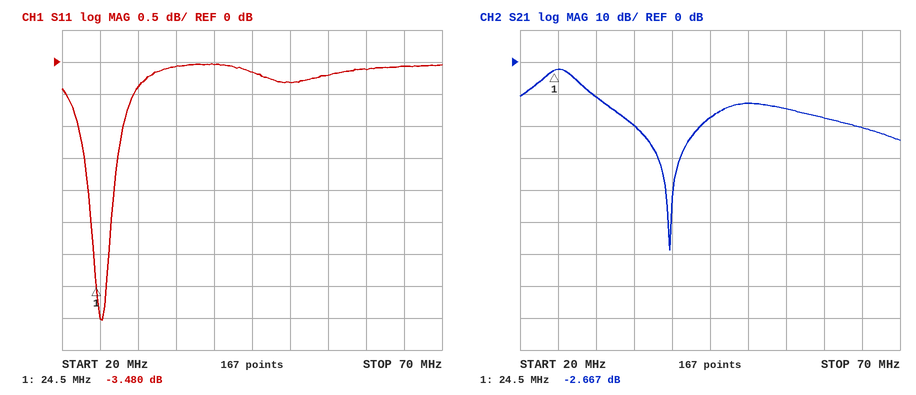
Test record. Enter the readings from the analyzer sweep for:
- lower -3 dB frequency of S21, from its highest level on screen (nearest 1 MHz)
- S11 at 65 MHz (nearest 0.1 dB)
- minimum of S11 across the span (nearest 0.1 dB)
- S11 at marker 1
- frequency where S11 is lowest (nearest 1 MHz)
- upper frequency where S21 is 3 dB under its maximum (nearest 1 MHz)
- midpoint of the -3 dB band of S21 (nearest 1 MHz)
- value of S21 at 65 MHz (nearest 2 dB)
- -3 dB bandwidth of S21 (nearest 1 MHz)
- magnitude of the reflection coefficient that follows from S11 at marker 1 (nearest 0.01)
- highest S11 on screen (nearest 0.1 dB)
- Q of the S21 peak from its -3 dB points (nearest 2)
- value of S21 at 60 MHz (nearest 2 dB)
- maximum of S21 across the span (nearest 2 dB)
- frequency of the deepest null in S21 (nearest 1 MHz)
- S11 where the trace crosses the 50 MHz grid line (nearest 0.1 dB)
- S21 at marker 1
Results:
23 MHz
-0.1 dB
-4.0 dB
-3.480 dB
25 MHz
27 MHz
25 MHz
-20 dB
4 MHz
0.67
0.0 dB
6
-18 dB
-2 dB
40 MHz
-0.3 dB
-2.667 dB
